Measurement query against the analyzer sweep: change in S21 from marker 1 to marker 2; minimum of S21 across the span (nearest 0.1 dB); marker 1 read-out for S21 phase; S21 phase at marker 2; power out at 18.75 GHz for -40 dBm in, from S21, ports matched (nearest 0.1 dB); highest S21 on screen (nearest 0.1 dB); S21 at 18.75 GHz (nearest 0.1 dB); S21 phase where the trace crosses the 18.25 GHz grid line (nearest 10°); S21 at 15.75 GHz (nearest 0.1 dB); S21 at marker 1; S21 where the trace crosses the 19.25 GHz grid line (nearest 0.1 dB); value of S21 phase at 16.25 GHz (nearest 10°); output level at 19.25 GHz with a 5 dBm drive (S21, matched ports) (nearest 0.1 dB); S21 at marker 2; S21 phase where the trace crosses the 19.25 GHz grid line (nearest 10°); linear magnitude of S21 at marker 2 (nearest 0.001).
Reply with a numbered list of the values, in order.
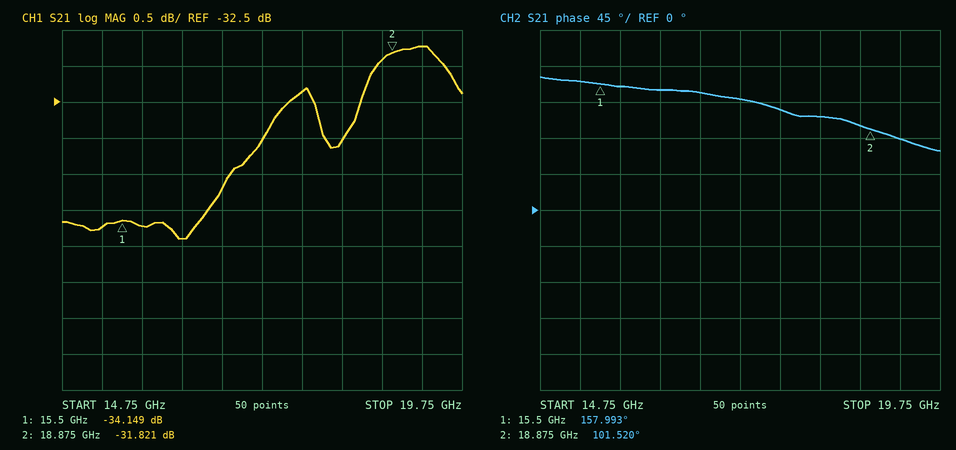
1. 2.328 dB
2. -34.4 dB
3. 157.993°
4. 101.520°
5. -71.9 dBm
6. -31.7 dB
7. -31.9 dB
8. 120°
9. -34.2 dB
10. -34.149 dB
11. -31.7 dB
12. 150°
13. -26.7 dBm
14. -31.821 dB
15. 90°
16. 0.026
